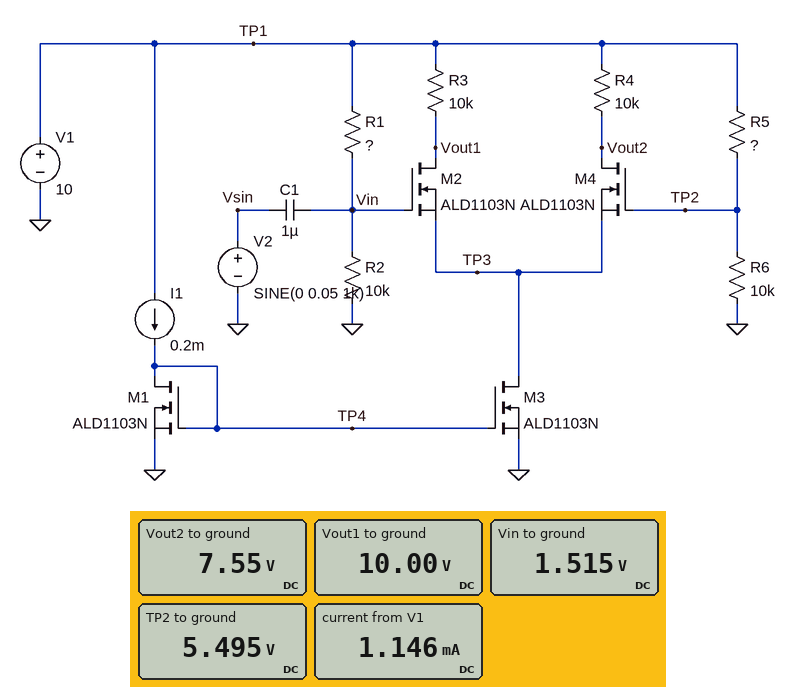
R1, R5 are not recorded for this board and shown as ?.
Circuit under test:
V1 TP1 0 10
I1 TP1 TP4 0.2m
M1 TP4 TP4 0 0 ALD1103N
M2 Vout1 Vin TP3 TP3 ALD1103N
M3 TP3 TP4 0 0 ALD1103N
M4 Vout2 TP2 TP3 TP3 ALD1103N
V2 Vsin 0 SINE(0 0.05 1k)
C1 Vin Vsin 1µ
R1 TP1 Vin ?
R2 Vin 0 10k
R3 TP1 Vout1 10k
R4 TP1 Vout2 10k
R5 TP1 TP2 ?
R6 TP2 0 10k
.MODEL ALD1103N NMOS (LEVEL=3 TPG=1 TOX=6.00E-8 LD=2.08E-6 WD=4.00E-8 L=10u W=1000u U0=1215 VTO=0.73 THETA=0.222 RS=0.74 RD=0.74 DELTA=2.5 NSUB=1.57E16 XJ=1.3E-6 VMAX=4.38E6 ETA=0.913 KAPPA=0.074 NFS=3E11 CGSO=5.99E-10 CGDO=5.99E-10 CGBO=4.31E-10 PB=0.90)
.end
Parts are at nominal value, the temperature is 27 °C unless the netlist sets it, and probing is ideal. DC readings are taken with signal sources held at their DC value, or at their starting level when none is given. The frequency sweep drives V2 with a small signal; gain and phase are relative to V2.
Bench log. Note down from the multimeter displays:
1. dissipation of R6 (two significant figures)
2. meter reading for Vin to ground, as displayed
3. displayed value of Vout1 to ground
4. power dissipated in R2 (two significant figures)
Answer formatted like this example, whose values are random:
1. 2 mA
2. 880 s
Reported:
1. 3.0 mW
2. 1.515 V
3. 10.00 V
4. 230 µW
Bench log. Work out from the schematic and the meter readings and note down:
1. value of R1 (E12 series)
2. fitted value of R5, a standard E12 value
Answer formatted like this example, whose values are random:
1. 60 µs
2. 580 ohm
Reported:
1. 56 kΩ
2. 8.2 kΩ
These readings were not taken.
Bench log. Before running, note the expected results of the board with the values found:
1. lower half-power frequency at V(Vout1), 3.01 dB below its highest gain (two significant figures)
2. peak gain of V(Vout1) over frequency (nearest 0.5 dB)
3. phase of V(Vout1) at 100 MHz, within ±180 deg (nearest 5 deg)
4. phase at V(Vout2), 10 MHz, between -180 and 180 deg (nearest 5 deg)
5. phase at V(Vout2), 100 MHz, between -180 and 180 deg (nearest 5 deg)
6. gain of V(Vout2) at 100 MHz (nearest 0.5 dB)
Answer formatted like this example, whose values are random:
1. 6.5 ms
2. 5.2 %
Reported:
1. 27 MHz
2. 0 dB
3. 15 deg
4. 20 deg
5. -5 deg
6. -5.5 dB
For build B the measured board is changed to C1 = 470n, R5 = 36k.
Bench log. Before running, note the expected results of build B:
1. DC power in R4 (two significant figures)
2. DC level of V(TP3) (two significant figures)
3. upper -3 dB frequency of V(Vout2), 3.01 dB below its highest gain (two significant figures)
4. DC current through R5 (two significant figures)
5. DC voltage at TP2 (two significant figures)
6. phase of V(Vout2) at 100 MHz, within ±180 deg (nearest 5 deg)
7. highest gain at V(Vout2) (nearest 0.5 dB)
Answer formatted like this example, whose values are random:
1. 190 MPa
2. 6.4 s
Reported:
1. 420 µW
2. 1.3 V
3. 15 MHz
4. 220 µA
5. 2.2 V
6. 5 deg
7. 5.5 dB
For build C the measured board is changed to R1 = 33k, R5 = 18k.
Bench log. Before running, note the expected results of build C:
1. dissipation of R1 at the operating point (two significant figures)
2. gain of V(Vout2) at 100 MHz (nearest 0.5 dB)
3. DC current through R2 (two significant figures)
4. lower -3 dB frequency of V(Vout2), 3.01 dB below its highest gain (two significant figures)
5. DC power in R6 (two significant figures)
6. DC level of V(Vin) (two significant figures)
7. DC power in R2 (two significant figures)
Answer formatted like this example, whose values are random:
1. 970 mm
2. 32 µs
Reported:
1. 1.8 mW
2. -4.5 dB
3. 230 µA
4. 6.2 MHz
5. 1.3 mW
6. 2.3 V
7. 540 µW
